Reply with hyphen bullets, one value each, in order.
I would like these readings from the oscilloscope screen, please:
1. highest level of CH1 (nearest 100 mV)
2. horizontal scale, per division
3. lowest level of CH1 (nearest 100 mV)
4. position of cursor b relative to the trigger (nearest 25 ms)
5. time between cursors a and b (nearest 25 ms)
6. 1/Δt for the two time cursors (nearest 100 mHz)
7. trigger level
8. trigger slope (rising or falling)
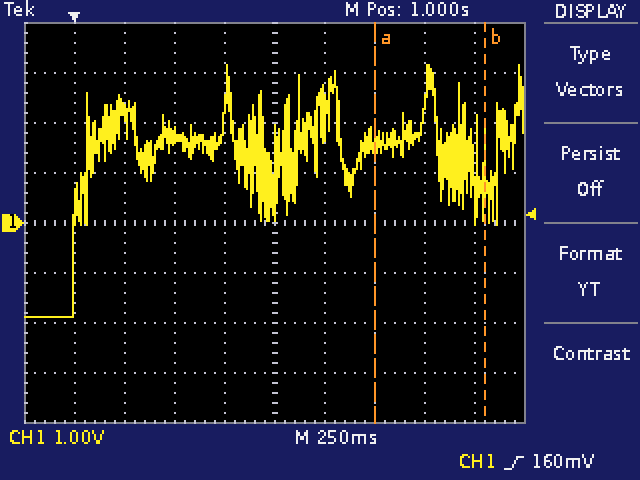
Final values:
- 3.2 V
- 250 ms
- -1.9 V
- +2.050 s
- 550 ms
- 1.8 Hz
- 160 mV
- rising
